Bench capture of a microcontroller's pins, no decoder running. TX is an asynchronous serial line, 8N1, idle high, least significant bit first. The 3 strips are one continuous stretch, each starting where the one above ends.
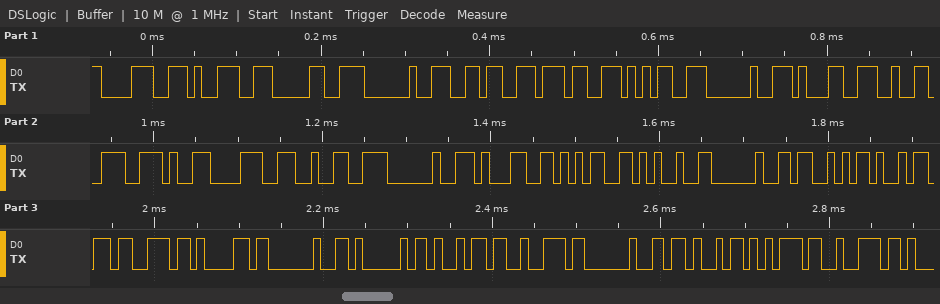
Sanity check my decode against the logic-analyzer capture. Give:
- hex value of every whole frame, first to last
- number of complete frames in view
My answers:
38 39 30 20 36 37 35 20 31 32 2E 38 32 20 31 35 25 20 53 69 73 61 20 41 69 72 20 4B 75 72
30
